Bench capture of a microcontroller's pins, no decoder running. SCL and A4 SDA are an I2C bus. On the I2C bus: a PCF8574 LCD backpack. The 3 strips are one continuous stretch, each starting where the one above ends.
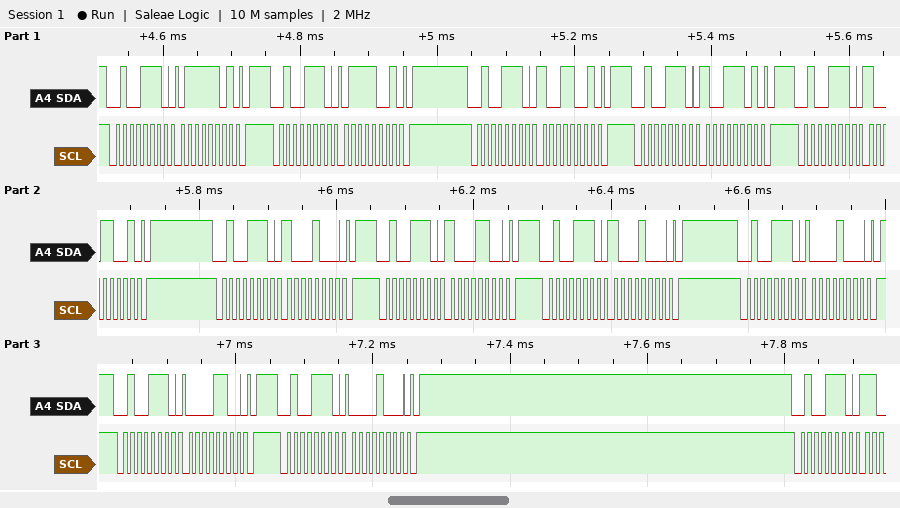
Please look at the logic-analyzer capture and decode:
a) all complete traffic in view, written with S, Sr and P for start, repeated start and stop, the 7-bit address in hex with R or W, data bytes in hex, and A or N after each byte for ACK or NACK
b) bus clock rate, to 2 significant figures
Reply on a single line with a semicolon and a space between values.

S 27W A 7D A P S 27W A 79 A P S 27W A 99 A P S 27W A 9D A P S 27W A 99 A P S 27W A 88 A P S 27W A 8C A P S 27W A 88 A P S 27W A 08 A P S 27W A 0C A P S 27W A 08 A P S 27W A; 100 kHz
